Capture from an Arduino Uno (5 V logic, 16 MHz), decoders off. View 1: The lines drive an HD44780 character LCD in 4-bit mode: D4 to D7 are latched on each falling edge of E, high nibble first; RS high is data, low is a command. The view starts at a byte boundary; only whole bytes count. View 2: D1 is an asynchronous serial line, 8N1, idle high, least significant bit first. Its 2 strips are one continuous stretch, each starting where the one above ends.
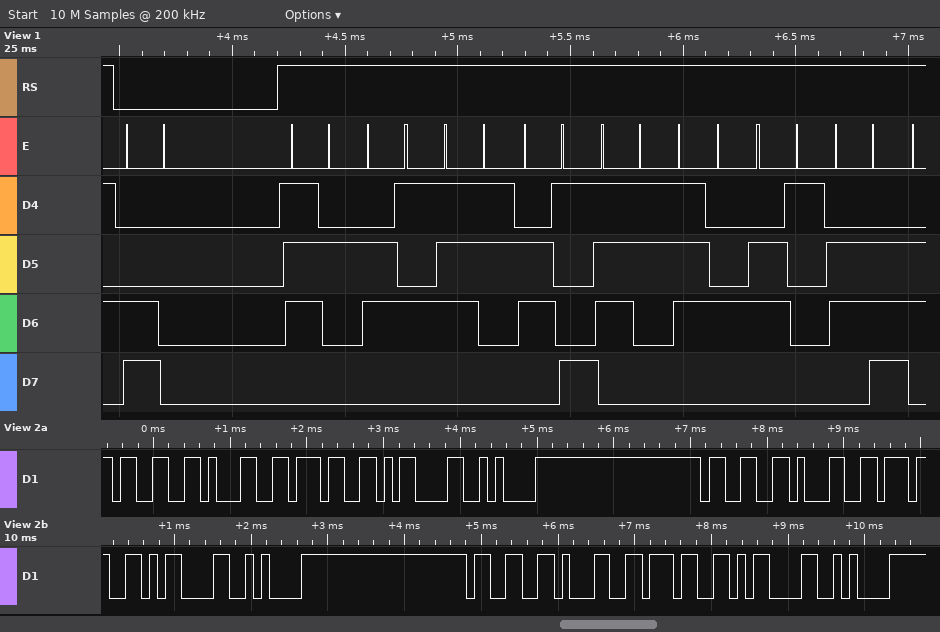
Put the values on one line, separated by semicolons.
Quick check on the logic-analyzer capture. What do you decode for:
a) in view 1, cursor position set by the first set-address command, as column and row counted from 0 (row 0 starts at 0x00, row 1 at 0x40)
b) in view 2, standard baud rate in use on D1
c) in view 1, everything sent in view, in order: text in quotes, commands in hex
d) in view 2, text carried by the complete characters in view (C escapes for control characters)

column 0, row 1; 9600 baud; 0xC0 "resistan"; "317\r\n317\r\n317\r\n"
